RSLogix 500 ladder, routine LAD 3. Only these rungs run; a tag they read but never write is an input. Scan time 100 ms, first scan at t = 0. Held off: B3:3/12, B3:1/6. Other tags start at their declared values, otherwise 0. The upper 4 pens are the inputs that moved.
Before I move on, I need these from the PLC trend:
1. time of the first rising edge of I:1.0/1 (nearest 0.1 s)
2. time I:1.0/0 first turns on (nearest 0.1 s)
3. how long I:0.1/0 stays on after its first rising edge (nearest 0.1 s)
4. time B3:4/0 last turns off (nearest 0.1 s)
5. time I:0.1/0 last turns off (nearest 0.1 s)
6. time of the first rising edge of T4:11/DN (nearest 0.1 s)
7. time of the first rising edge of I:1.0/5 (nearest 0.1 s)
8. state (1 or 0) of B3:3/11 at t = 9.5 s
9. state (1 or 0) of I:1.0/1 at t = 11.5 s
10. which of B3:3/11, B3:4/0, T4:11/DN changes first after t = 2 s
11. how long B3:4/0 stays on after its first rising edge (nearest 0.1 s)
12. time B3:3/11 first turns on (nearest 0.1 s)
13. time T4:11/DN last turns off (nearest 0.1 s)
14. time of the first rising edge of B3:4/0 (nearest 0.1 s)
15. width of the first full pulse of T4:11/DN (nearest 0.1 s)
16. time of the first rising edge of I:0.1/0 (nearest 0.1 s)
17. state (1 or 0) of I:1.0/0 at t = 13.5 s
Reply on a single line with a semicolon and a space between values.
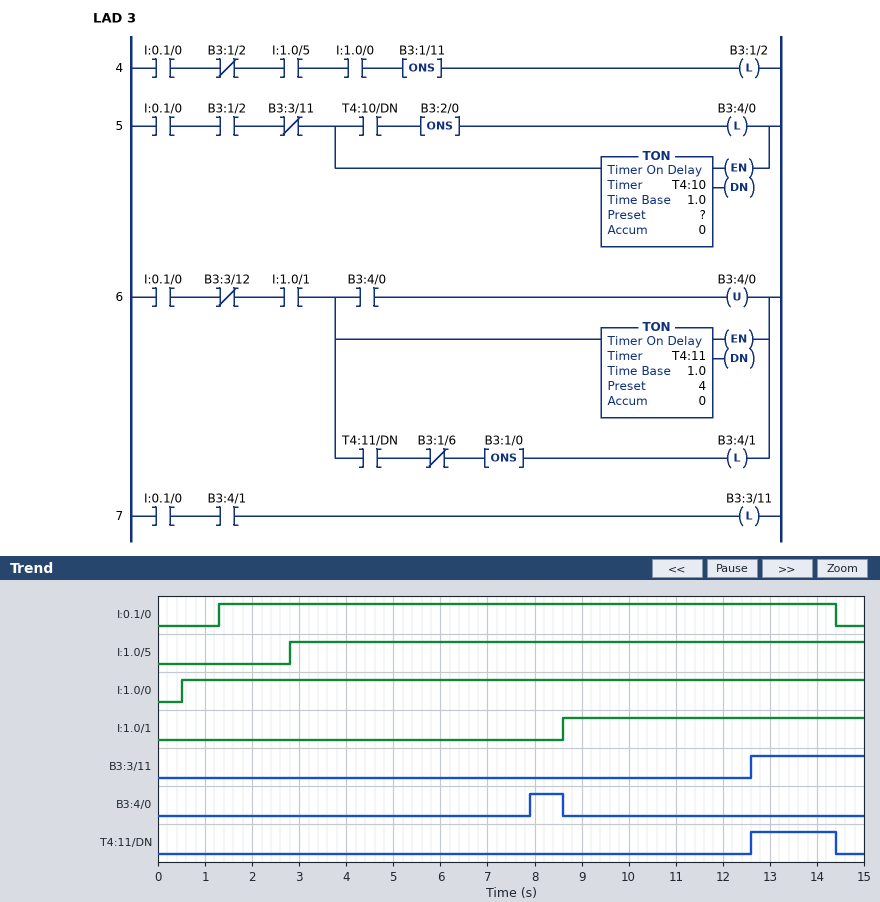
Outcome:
8.6 s; 0.5 s; 13.1 s; 8.6 s; 14.4 s; 12.6 s; 2.8 s; 0; 1; B3:4/0; 0.7 s; 12.6 s; 14.4 s; 7.9 s; 1.8 s; 1.3 s; 1
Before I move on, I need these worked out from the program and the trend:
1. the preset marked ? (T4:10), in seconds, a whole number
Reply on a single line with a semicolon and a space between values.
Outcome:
5 s
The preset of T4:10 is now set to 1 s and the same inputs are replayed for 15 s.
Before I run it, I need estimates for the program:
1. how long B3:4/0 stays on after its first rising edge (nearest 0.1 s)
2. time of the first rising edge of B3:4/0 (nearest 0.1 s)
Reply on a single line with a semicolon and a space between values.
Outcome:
4.7 s; 3.9 s
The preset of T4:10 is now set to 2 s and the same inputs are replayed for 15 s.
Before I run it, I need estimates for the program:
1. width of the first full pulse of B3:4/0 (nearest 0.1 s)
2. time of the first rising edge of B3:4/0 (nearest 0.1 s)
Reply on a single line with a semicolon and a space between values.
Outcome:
3.7 s; 4.9 s
